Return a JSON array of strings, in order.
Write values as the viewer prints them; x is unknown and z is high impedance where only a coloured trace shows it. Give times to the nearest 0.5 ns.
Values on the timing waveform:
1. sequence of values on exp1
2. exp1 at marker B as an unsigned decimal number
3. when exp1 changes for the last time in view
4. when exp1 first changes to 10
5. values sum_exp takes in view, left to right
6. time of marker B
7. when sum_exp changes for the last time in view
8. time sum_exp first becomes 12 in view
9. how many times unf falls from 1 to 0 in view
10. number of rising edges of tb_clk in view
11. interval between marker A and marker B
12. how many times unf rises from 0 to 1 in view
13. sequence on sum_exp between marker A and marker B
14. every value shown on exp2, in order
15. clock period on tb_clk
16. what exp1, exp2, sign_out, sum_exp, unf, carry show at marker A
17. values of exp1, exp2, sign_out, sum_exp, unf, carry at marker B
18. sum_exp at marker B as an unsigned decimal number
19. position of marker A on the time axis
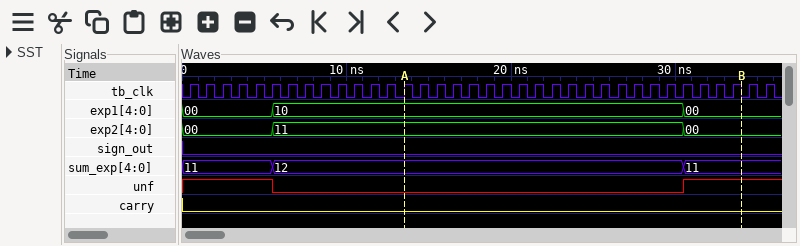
["00, 10, 00", "0", "30.5 ns", "5.5 ns", "11, 12, 11", "34 ns", "30.5 ns", "5.5 ns", "1", "36", "20.5 ns", "1", "12, 11", "00, 11, 00", "1 ns", "exp1=10, exp2=11, sign_out=0, sum_exp=12, unf=0, carry=0", "exp1=00, exp2=00, sign_out=0, sum_exp=11, unf=1, carry=0", "17", "13.5 ns"]
